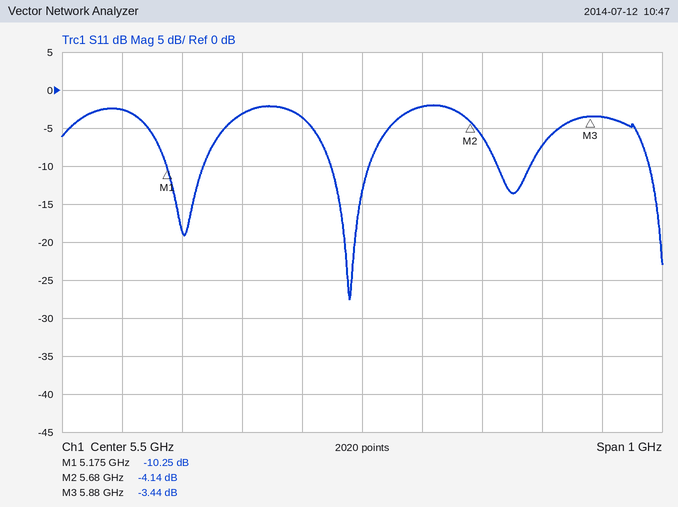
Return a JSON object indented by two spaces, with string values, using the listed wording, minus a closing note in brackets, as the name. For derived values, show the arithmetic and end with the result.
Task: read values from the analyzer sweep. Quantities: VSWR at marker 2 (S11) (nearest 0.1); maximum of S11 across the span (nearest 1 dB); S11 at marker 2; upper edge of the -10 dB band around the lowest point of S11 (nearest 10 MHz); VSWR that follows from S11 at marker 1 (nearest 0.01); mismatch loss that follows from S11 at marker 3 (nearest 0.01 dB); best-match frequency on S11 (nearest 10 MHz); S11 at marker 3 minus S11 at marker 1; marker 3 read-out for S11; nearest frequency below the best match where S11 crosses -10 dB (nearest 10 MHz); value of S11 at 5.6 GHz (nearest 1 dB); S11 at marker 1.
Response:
{
  "VSWR at marker 2 (S11)": "(1 + 0.6209)/(1 − 0.6209) ≈ 4.3",
  "maximum of S11 across the span": "-2 dB",
  "S11 at marker 2": "-4.14 dB",
  "upper edge of the -10 dB band around the lowest point of S11": "5.51 GHz",
  "VSWR that follows from S11 at marker 1": "(1 + 0.3073)/(1 − 0.3073) ≈ 1.89",
  "mismatch loss that follows from S11 at marker 3": "−10 log10(1 − 10^(-3.44/10)) ≈ 2.62 dB",
  "best-match frequency on S11": "5.48 GHz",
  "S11 at marker 3 minus S11 at marker 1": "-3.44 − (-10.25) = 6.81 dB",
  "marker 3 read-out for S11": "-3.44 dB",
  "nearest frequency below the best match where S11 crosses -10 dB": "5.45 GHz",
  "value of S11 at 5.6 GHz": "-2 dB",
  "S11 at marker 1": "-10.25 dB"
}
